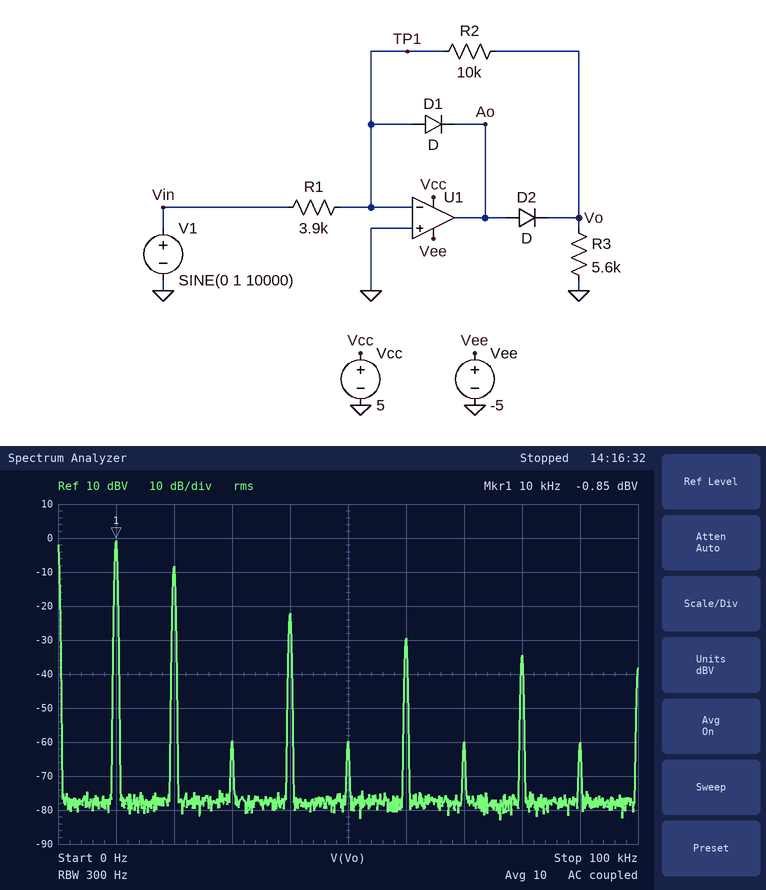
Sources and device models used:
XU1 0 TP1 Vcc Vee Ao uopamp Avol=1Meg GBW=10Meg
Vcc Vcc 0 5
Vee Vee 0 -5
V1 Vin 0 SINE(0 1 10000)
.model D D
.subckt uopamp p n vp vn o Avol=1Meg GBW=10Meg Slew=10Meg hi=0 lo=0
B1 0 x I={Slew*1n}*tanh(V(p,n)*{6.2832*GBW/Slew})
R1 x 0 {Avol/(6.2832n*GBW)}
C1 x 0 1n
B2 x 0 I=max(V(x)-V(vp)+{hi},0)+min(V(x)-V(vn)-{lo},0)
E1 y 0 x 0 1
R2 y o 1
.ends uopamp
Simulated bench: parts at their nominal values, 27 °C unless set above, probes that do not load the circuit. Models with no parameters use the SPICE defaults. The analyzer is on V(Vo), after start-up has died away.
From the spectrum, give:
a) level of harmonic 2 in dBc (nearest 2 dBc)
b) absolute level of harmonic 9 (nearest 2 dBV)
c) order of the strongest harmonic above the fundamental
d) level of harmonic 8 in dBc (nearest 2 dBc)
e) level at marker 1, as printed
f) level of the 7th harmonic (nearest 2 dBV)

-8 dBc
-60 dBV
2
-34 dBc
-0.85 dBV
-60 dBV
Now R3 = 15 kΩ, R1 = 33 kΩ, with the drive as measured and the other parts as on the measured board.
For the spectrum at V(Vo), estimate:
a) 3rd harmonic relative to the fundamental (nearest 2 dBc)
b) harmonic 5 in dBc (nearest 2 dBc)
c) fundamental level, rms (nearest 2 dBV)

-48 dBc
-48 dBc
-20 dBV
